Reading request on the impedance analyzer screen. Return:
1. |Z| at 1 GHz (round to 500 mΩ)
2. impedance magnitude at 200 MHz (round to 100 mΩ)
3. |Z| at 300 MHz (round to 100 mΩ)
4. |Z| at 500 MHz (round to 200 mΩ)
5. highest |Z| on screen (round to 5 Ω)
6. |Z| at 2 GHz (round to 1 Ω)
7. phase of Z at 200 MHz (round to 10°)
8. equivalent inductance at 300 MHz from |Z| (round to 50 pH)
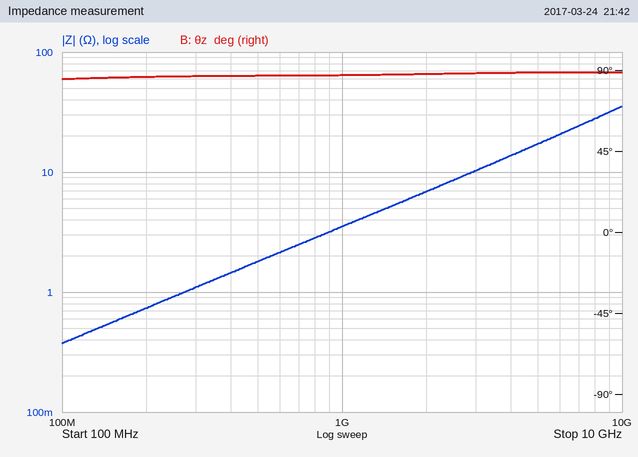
3.5 Ω
700 mΩ
1.1 Ω
1.8 Ω
35 Ω
7 Ω
90°
600 pH
